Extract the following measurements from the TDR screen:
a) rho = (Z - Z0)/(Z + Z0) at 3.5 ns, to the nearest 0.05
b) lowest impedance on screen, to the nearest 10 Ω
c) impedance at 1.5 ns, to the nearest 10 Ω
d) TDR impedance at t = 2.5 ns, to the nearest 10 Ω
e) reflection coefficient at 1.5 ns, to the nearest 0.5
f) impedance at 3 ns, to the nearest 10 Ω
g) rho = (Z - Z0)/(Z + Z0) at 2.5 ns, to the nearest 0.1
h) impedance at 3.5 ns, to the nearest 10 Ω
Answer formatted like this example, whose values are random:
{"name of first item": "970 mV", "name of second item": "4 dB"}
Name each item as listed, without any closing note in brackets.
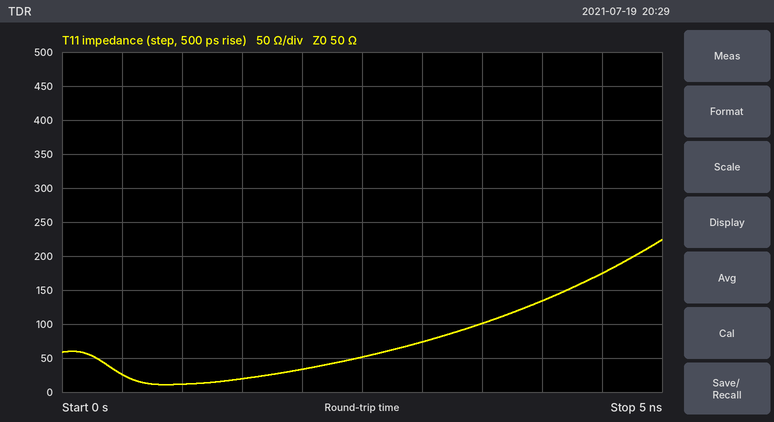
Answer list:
{"rho = (Z - Z0)/(Z + Z0) at 3.5 ns, to the nearest 0.05": "+0.35", "lowest impedance on screen, to the nearest 10 Ω": "10 Ω", "impedance at 1.5 ns, to the nearest 10 Ω": "20 Ω", "TDR impedance at t = 2.5 ns, to the nearest 10 Ω": "50 Ω", "reflection coefficient at 1.5 ns, to the nearest 0.5": "-0.5", "impedance at 3 ns, to the nearest 10 Ω": "70 Ω", "rho = (Z - Z0)/(Z + Z0) at 2.5 ns, to the nearest 0.1": "0.0", "impedance at 3.5 ns, to the nearest 10 Ω": "100 Ω"}
